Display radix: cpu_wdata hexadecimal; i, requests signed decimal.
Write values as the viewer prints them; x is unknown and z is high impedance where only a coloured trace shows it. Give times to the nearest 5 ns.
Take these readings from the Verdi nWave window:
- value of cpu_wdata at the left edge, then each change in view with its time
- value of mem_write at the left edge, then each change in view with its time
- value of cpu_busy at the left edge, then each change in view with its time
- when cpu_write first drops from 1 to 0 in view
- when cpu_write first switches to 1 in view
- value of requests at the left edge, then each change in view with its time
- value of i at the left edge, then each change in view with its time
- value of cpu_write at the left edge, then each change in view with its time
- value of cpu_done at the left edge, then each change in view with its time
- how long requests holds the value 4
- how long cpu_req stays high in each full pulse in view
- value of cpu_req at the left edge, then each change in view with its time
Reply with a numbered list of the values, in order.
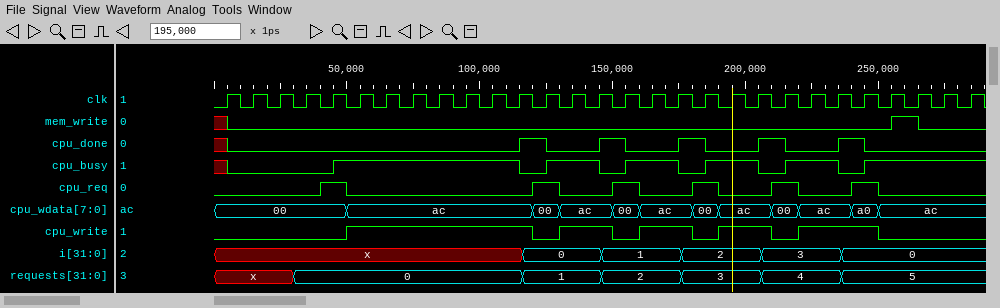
1. 00, ac at 50 ns, 00 at 120 ns, ac at 130 ns, 00 at 150 ns, ac at 160 ns, 00 at 180 ns, ac at 190 ns, 00 at 210 ns, ac at 220 ns, a0 at 240 ns, ac at 250 ns
2. x, 0 at 5 ns, 1 at 255 ns, 0 at 265 ns
3. x, 0 at 5 ns, 1 at 45 ns, 0 at 115 ns, 1 at 125 ns, 0 at 145 ns, 1 at 155 ns, 0 at 175 ns, 1 at 185 ns, 0 at 205 ns, 1 at 215 ns, 0 at 235 ns, 1 at 245 ns
4. 120 ns
5. 50 ns
6. x, 0 at 30 ns, 1 at 115 ns, 2 at 145 ns, 3 at 175 ns, 4 at 205 ns, 5 at 235 ns
7. x, 0 at 115 ns, 1 at 145 ns, 2 at 175 ns, 3 at 205 ns, 0 at 235 ns
8. 0, 1 at 50 ns, 0 at 120 ns, 1 at 130 ns, 0 at 150 ns, 1 at 160 ns, 0 at 180 ns, 1 at 190 ns, 0 at 210 ns, 1 at 220 ns, 0 at 250 ns
9. x, 0 at 5 ns, 1 at 115 ns, 0 at 125 ns, 1 at 145 ns, 0 at 155 ns, 1 at 175 ns, 0 at 185 ns, 1 at 205 ns, 0 at 215 ns, 1 at 235 ns, 0 at 245 ns
10. 30 ns
11. 10 ns, 10 ns, 10 ns, 10 ns, 10 ns, 10 ns
12. 0, 1 at 40 ns, 0 at 50 ns, 1 at 120 ns, 0 at 130 ns, 1 at 150 ns, 0 at 160 ns, 1 at 180 ns, 0 at 190 ns, 1 at 210 ns, 0 at 220 ns, 1 at 240 ns, 0 at 250 ns
